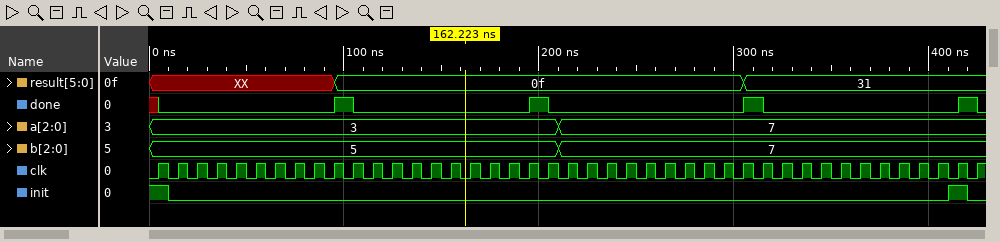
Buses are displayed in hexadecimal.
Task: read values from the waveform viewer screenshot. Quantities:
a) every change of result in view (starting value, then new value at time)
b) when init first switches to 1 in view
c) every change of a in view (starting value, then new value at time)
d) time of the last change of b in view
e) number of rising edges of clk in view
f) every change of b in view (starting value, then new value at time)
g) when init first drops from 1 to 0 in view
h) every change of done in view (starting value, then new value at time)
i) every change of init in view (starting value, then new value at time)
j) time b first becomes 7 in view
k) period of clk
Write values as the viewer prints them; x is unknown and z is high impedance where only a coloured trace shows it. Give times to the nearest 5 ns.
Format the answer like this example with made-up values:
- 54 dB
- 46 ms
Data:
- XX, 0f at 95 ns, 31 at 305 ns
- 410 ns
- 3, 7 at 210 ns
- 210 ns
- 43
- 5, 7 at 210 ns
- 10 ns
- x, 0 at 5 ns, 1 at 95 ns, 0 at 105 ns, 1 at 195 ns, 0 at 205 ns, 1 at 305 ns, 0 at 315 ns, 1 at 415 ns, 0 at 425 ns
- 1, 0 at 10 ns, 1 at 410 ns, 0 at 420 ns
- 210 ns
- 10 ns
